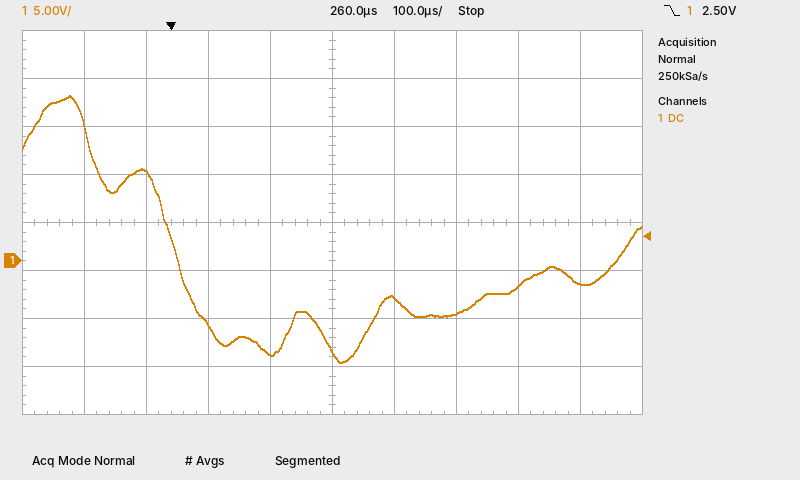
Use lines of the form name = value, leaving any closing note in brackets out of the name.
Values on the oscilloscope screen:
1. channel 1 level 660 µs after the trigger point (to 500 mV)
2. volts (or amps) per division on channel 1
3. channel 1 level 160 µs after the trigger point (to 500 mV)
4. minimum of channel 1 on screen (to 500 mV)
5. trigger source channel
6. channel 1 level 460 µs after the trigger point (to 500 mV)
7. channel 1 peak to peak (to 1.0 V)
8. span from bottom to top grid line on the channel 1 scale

channel 1 level 660 µs after the trigger point = -2.5 V
volts (or amps) per division on channel 1 = 5 V
channel 1 level 160 µs after the trigger point = -9.5 V
minimum of channel 1 on screen = -10.5 V
trigger source channel = channel 1
channel 1 level 460 µs after the trigger point = -5.5 V
channel 1 peak to peak = 28.0 V
span from bottom to top grid line on the channel 1 scale = 40 V
